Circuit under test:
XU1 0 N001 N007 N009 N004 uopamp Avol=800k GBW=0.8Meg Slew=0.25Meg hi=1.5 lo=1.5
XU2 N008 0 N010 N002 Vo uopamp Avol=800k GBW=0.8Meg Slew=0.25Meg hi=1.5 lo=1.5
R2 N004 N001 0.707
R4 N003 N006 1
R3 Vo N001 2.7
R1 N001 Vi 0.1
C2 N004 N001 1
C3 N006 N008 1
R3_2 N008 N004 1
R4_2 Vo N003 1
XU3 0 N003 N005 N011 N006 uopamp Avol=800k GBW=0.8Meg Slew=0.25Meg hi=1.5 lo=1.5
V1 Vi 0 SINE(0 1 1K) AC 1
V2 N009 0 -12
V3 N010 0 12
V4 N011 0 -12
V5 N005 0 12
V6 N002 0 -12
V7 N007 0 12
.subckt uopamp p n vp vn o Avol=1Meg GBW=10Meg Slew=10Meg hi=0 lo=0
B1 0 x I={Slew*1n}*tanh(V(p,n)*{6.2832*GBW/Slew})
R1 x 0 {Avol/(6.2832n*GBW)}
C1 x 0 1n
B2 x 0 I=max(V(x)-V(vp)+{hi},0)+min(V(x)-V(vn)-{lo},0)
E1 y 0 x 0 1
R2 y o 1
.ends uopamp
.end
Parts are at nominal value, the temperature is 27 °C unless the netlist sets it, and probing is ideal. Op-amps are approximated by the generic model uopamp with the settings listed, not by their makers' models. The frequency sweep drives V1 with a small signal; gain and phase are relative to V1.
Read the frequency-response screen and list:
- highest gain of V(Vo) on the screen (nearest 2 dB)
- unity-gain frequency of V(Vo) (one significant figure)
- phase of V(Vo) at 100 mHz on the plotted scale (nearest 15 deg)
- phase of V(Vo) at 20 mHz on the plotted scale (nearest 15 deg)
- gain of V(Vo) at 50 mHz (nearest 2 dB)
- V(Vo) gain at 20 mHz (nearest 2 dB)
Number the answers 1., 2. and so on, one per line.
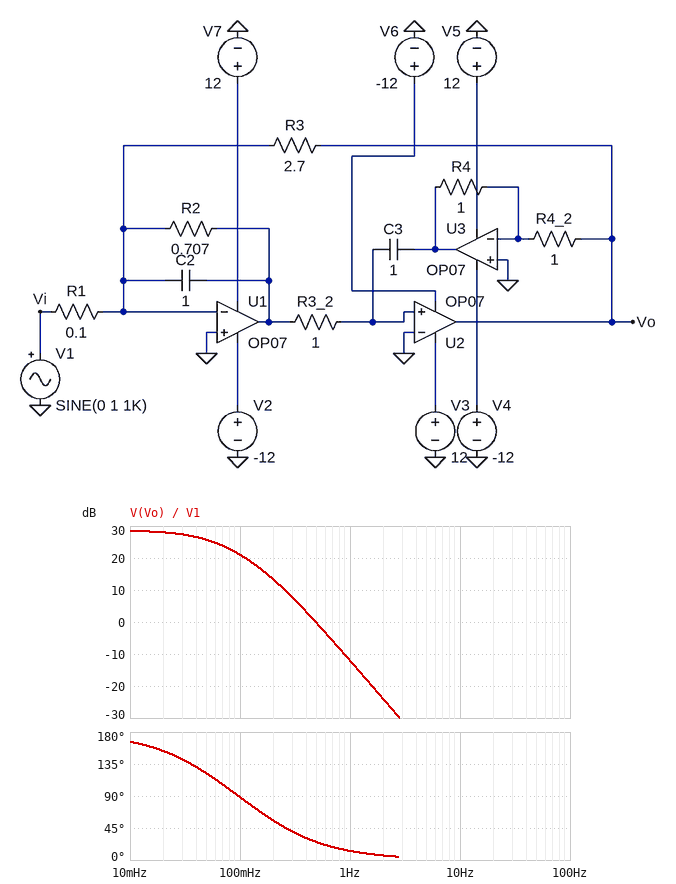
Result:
1. 28 dB
2. 500 mHz
3. 90 deg
4. 150 deg
5. 26 dB
6. 28 dB
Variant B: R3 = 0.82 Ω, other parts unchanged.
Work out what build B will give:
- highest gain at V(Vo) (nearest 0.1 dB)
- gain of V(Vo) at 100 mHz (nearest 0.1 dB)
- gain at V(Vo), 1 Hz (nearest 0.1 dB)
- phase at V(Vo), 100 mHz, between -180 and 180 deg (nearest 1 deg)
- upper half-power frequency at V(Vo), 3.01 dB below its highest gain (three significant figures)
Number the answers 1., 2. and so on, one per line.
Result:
1. 18.4 dB
2. 18.3 dB
3. -11.9 dB
4. 133 deg
5. 190 mHz
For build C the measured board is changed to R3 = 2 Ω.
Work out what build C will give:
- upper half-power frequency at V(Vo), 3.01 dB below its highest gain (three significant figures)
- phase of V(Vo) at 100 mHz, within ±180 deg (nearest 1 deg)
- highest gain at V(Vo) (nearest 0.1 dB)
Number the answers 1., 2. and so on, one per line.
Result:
1. 72.4 mHz
2. 97 deg
3. 26.0 dB
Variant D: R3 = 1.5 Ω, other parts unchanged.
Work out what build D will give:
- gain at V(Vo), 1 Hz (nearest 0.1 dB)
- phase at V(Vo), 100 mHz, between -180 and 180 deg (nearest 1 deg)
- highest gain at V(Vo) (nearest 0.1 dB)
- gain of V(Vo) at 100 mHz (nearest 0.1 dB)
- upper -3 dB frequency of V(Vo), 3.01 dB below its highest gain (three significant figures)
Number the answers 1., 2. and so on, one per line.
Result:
1. -12.0 dB
2. 107 deg
3. 23.5 dB
4. 20.6 dB
5. 102 mHz
